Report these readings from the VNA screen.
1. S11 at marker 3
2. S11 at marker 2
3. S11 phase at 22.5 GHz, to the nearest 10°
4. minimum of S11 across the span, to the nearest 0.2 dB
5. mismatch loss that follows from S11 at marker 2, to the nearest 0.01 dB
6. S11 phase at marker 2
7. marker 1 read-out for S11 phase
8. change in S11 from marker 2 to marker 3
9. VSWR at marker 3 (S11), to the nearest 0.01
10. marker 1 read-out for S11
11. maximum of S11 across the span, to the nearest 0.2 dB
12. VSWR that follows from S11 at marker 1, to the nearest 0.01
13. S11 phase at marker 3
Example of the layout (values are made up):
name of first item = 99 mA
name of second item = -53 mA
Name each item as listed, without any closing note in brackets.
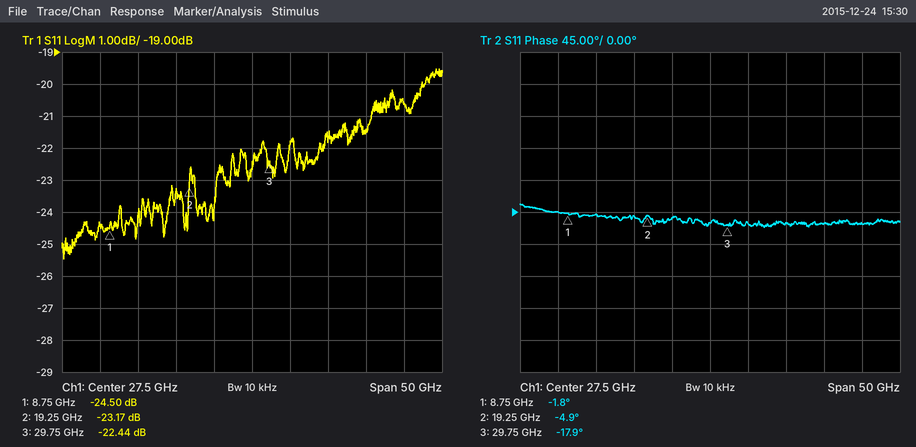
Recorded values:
S11 at marker 3 = -22.44 dB
S11 at marker 2 = -23.17 dB
S11 phase at 22.5 GHz, to the nearest 10° = -10°
minimum of S11 across the span, to the nearest 0.2 dB = -25.4 dB
mismatch loss that follows from S11 at marker 2, to the nearest 0.01 dB = 0.02 dB
S11 phase at marker 2 = -4.9°
marker 1 read-out for S11 phase = -1.8°
change in S11 from marker 2 to marker 3 = 0.73 dB
VSWR at marker 3 (S11), to the nearest 0.01 = 1.16
marker 1 read-out for S11 = -24.50 dB
maximum of S11 across the span, to the nearest 0.2 dB = -19.6 dB
VSWR that follows from S11 at marker 1, to the nearest 0.01 = 1.13
S11 phase at marker 3 = -17.9°
